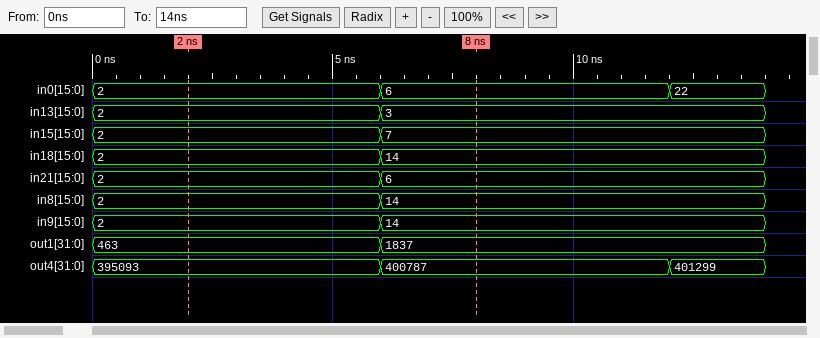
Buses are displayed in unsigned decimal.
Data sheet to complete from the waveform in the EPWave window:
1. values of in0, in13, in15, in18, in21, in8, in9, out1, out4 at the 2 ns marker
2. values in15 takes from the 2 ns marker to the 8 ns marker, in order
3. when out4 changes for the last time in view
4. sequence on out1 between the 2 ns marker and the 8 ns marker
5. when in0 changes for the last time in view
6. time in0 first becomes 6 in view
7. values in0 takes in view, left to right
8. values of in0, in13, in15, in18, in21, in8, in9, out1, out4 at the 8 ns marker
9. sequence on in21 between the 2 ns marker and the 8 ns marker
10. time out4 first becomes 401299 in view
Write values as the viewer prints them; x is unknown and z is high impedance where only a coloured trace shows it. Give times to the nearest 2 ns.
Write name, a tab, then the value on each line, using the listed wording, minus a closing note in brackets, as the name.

values of in0, in13, in15, in18, in21, in8, in9, out1, out4 at the 2 ns marker	in0=2, in13=2, in15=2, in18=2, in21=2, in8=2, in9=2, out1=463, out4=395093
values in15 takes from the 2 ns marker to the 8 ns marker, in order	2, 7
when out4 changes for the last time in view	12 ns
sequence on out1 between the 2 ns marker and the 8 ns marker	463, 1837
when in0 changes for the last time in view	12 ns
time in0 first becomes 6 in view	6 ns
values in0 takes in view, left to right	2, 6, 22
values of in0, in13, in15, in18, in21, in8, in9, out1, out4 at the 8 ns marker	in0=6, in13=3, in15=7, in18=14, in21=6, in8=14, in9=14, out1=1837, out4=400787
sequence on in21 between the 2 ns marker and the 8 ns marker	2, 6
time out4 first becomes 401299 in view	12 ns
